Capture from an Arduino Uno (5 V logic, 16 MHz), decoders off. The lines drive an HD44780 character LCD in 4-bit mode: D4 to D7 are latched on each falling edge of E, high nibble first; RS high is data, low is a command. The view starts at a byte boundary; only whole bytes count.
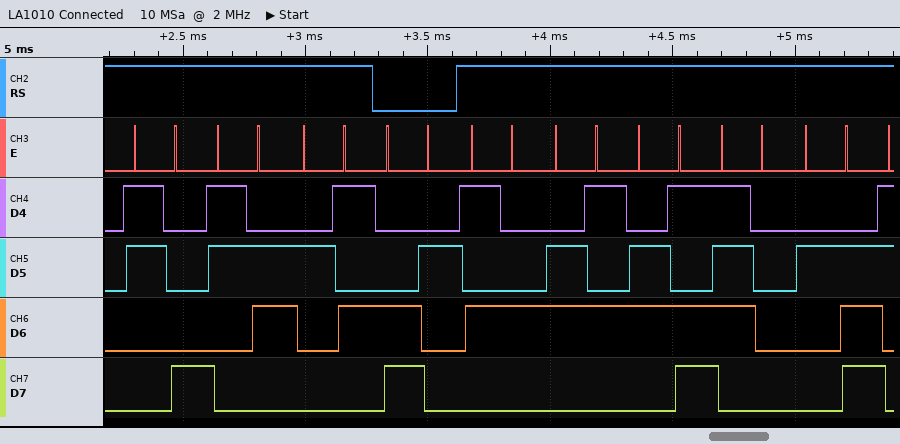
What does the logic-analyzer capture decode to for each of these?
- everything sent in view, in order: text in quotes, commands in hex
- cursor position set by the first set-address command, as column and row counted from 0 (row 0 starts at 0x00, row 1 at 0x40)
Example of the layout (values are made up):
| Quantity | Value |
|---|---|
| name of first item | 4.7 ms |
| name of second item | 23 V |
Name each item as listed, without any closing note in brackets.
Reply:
| Quantity | Value |
|---|---|
| everything sent in view, in order: text in quotes, commands in hex | "86%" 0xC2 "Temp." |
| cursor position set by the first set-address command, as column and row counted from 0 | column 2, row 1 |
